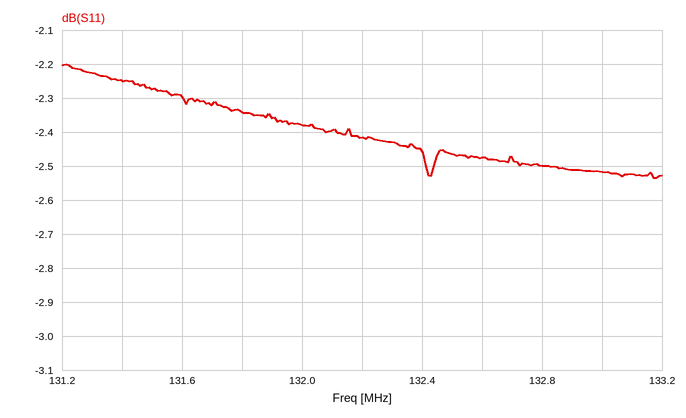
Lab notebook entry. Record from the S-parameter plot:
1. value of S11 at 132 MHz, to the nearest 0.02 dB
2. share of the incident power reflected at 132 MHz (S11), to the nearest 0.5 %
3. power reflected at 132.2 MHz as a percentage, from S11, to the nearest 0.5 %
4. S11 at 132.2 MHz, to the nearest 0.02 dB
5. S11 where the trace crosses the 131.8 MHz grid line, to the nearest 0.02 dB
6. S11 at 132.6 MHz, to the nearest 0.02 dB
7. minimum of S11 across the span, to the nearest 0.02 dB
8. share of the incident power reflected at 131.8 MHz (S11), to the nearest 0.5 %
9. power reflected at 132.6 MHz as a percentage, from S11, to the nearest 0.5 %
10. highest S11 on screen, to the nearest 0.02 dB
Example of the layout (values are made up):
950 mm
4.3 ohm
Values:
-2.38 dB
58.0 %
57.5 %
-2.42 dB
-2.34 dB
-2.48 dB
-2.54 dB
58.5 %
56.5 %
-2.20 dB
